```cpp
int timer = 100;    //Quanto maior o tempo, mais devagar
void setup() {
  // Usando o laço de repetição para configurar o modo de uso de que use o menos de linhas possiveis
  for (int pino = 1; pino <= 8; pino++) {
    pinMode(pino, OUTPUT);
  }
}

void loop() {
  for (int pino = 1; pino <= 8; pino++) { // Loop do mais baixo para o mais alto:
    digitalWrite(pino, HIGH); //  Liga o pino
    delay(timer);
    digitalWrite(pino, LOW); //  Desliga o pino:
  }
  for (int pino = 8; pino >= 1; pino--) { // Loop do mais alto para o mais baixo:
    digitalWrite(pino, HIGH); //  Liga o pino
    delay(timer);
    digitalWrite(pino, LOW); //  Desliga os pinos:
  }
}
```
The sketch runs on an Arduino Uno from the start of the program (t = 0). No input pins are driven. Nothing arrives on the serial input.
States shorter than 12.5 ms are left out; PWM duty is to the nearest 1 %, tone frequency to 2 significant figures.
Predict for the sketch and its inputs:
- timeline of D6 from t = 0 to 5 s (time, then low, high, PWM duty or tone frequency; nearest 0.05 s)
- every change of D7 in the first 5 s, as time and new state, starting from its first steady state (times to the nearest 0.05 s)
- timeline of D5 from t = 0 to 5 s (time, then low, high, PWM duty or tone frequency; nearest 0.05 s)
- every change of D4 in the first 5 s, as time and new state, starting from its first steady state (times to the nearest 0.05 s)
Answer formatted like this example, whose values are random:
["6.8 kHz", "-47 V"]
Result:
["0 s low; 0.5 s high; 0.6 s low; 1 s high; 1.1 s low; 2.1 s high; 2.2 s low; 2.6 s high; 2.7 s low; 3.7 s high; 3.8 s low; 4.2 s high; 4.3 s low", "0 s low; 0.6 s high; 0.7 s low; 0.9 s high; 1 s low; 2.2 s high; 2.3 s low; 2.5 s high; 2.6 s low; 3.8 s high; 3.9 s low; 4.1 s high; 4.2 s low", "0 s low; 0.4 s high; 0.5 s low; 1.1 s high; 1.2 s low; 2 s high; 2.1 s low; 2.7 s high; 2.8 s low; 3.6 s high; 3.7 s low; 4.3 s high; 4.4 s low", "0 s low; 0.3 s high; 0.4 s low; 1.2 s high; 1.3 s low; 1.9 s high; 2 s low; 2.8 s high; 2.9 s low; 3.5 s high; 3.6 s low; 4.4 s high; 4.5 s low"]
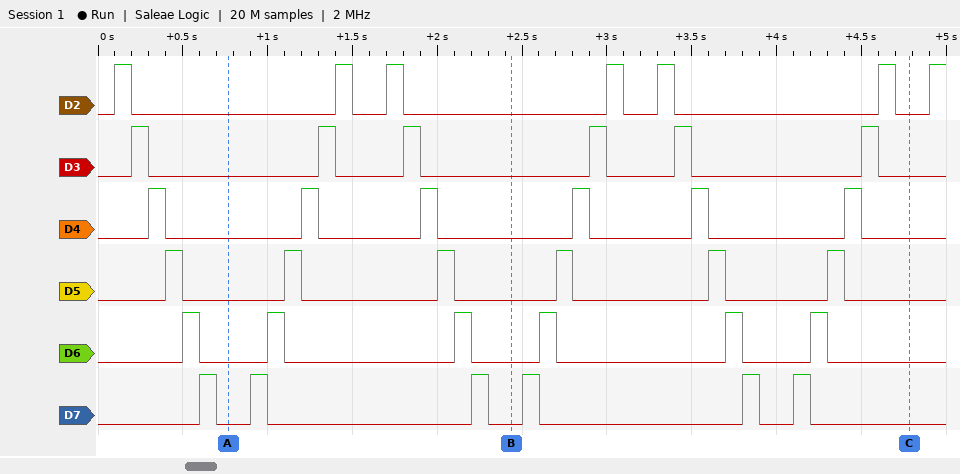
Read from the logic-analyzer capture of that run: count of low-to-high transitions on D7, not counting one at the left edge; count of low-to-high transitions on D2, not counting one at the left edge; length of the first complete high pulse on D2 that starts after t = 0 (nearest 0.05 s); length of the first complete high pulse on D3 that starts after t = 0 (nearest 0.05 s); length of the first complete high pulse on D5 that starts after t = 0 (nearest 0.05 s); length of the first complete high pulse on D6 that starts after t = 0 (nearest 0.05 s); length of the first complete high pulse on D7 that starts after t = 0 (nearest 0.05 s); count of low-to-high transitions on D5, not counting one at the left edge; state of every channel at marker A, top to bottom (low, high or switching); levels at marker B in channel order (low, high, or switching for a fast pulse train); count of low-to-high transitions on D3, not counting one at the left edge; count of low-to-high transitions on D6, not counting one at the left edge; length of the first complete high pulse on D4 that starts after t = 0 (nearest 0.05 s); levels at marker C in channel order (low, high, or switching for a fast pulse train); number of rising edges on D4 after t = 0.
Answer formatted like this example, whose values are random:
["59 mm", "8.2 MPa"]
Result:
["6", "7", "0.10 s", "0.10 s", "0.10 s", "0.10 s", "0.10 s", "6", "D2 low, D3 low, D4 low, D5 low, D6 low, D7 low", "D2 low, D3 low, D4 low, D5 low, D6 low, D7 low", "6", "6", "0.10 s", "D2 low, D3 low, D4 low, D5 low, D6 low, D7 low", "6"]
